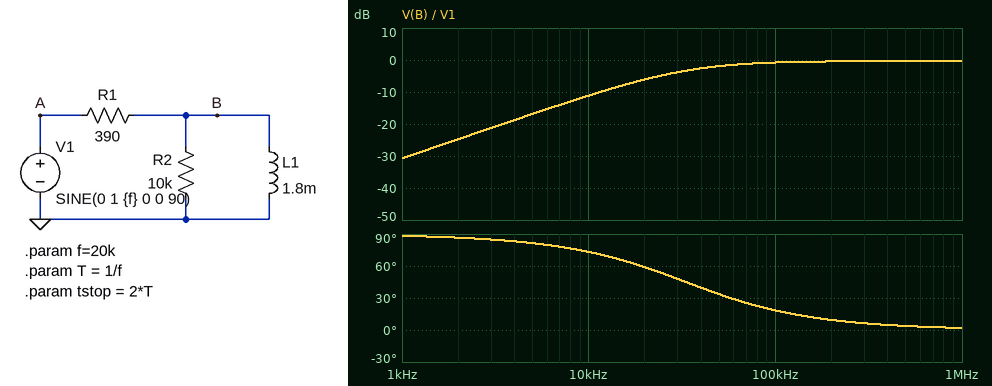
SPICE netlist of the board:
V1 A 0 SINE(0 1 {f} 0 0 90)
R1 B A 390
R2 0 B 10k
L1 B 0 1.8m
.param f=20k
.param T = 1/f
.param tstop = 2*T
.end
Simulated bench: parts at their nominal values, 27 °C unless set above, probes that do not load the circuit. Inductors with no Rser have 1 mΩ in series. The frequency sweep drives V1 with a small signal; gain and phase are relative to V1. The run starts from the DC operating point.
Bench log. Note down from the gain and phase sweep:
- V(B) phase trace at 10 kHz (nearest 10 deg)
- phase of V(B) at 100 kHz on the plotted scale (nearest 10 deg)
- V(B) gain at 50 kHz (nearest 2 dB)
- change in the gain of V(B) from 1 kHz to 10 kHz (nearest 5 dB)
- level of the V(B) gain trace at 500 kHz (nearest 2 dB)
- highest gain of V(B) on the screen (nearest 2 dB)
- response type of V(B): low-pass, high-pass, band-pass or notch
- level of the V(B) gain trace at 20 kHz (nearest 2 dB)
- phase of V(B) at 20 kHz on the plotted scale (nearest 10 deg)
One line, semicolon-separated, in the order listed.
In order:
70 deg; 20 deg; -2 dB; 20 dB; 0 dB; 0 dB; high-pass; -6 dB; 60 deg
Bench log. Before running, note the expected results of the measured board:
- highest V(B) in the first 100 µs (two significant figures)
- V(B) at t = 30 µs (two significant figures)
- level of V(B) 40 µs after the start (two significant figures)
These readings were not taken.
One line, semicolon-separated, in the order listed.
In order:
500 mV; 42 mV; 480 mV
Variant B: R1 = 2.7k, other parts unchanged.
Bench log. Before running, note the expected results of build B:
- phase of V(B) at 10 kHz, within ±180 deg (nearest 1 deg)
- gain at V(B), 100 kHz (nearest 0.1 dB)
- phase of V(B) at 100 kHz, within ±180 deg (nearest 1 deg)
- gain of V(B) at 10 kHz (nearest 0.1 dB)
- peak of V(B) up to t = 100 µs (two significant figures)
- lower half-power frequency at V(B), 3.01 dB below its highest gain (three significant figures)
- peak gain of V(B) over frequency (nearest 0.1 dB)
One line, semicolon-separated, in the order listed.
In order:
87 deg; -8.6 dB; 62 deg; -27.6 dB; 83 mV; 188 kHz; -2.1 dB
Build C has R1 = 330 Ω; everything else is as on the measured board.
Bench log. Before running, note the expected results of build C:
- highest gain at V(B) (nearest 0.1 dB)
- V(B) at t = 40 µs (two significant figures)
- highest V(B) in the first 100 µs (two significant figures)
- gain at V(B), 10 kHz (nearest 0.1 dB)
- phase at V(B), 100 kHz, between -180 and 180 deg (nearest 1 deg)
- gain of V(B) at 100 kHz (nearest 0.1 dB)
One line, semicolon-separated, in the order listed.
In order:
-0.3 dB; 530 mV; 560 mV; -9.8 dB; 16 deg; -0.6 dB
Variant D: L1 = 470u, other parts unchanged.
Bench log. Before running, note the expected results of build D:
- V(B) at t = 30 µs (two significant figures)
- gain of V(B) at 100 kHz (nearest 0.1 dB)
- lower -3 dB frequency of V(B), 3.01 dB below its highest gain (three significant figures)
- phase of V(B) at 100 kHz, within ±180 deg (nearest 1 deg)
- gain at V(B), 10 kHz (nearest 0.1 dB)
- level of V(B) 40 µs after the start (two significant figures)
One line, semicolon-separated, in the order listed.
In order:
68 mV; -4.5 dB; 127 kHz; 52 deg; -22.4 dB; 150 mV
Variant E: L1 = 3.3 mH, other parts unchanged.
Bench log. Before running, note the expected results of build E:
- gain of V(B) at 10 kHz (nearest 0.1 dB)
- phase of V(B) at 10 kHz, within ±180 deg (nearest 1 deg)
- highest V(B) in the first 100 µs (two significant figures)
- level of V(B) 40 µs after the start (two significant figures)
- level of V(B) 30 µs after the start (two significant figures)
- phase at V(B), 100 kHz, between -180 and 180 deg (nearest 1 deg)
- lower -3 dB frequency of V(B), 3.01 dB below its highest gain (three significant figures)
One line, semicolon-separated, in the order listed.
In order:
-6.6 dB; 61 deg; 710 mV; 610 mV; -160 mV; 10 deg; 18.1 kHz
